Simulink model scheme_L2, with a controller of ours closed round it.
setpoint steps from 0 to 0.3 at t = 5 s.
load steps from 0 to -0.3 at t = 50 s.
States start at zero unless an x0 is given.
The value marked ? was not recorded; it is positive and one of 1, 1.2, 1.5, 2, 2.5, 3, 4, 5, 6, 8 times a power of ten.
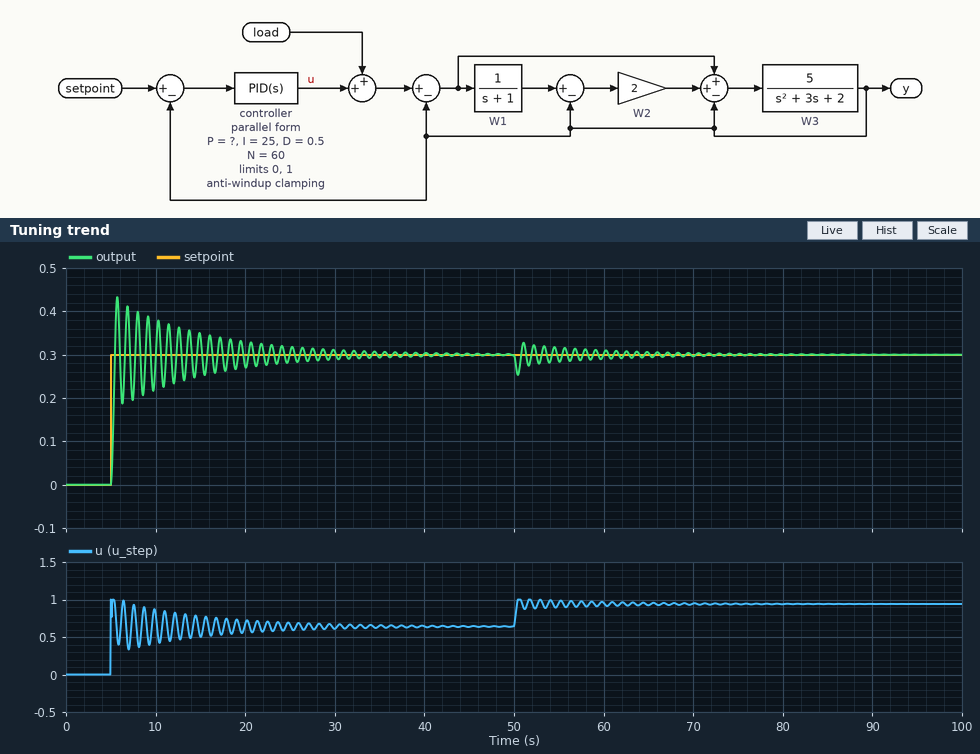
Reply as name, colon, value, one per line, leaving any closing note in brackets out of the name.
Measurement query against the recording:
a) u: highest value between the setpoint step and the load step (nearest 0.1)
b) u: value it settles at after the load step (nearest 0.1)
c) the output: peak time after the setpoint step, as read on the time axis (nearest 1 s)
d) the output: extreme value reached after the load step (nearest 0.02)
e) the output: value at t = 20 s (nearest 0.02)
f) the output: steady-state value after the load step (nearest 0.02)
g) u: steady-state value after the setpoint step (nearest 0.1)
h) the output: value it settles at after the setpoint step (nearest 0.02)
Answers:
u: highest value between the setpoint step and the load step: 1.0
u: value it settles at after the load step: 0.9
the output: peak time after the setpoint step, as read on the time axis: 6 s
the output: extreme value reached after the load step: 0.26
the output: value at t = 20 s: 0.28
the output: steady-state value after the load step: 0.30
u: steady-state value after the setpoint step: 0.6
the output: value it settles at after the setpoint step: 0.30
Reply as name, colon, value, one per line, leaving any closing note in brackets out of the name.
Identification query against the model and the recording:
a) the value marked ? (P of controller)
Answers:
the value marked ?: 2
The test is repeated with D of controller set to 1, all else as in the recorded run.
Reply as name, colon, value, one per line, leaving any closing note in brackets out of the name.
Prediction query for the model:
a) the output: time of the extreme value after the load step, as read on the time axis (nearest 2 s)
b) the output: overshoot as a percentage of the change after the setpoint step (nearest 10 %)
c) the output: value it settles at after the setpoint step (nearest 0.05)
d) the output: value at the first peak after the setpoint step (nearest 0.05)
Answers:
the output: time of the extreme value after the load step, as read on the time axis: 50 s
the output: overshoot as a percentage of the change after the setpoint step: 50 %
the output: value it settles at after the setpoint step: 0.30
the output: value at the first peak after the setpoint step: 0.45
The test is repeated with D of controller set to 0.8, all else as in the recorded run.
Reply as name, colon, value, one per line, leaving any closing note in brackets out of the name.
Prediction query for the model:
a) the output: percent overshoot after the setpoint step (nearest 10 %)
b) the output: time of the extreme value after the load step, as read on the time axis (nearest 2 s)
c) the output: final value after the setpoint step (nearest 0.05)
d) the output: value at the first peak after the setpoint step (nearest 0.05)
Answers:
the output: percent overshoot after the setpoint step: 50 %
the output: time of the extreme value after the load step, as read on the time axis: 50 s
the output: final value after the setpoint step: 0.30
the output: value at the first peak after the setpoint step: 0.45
